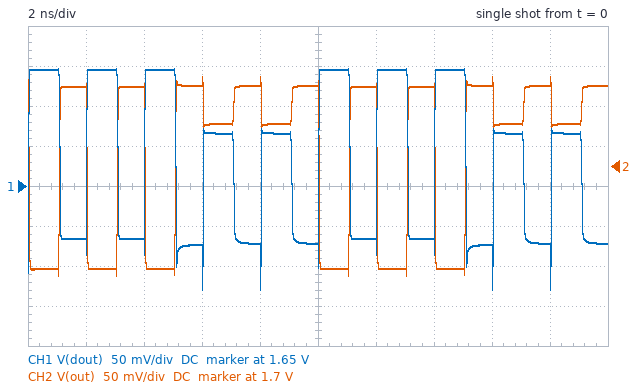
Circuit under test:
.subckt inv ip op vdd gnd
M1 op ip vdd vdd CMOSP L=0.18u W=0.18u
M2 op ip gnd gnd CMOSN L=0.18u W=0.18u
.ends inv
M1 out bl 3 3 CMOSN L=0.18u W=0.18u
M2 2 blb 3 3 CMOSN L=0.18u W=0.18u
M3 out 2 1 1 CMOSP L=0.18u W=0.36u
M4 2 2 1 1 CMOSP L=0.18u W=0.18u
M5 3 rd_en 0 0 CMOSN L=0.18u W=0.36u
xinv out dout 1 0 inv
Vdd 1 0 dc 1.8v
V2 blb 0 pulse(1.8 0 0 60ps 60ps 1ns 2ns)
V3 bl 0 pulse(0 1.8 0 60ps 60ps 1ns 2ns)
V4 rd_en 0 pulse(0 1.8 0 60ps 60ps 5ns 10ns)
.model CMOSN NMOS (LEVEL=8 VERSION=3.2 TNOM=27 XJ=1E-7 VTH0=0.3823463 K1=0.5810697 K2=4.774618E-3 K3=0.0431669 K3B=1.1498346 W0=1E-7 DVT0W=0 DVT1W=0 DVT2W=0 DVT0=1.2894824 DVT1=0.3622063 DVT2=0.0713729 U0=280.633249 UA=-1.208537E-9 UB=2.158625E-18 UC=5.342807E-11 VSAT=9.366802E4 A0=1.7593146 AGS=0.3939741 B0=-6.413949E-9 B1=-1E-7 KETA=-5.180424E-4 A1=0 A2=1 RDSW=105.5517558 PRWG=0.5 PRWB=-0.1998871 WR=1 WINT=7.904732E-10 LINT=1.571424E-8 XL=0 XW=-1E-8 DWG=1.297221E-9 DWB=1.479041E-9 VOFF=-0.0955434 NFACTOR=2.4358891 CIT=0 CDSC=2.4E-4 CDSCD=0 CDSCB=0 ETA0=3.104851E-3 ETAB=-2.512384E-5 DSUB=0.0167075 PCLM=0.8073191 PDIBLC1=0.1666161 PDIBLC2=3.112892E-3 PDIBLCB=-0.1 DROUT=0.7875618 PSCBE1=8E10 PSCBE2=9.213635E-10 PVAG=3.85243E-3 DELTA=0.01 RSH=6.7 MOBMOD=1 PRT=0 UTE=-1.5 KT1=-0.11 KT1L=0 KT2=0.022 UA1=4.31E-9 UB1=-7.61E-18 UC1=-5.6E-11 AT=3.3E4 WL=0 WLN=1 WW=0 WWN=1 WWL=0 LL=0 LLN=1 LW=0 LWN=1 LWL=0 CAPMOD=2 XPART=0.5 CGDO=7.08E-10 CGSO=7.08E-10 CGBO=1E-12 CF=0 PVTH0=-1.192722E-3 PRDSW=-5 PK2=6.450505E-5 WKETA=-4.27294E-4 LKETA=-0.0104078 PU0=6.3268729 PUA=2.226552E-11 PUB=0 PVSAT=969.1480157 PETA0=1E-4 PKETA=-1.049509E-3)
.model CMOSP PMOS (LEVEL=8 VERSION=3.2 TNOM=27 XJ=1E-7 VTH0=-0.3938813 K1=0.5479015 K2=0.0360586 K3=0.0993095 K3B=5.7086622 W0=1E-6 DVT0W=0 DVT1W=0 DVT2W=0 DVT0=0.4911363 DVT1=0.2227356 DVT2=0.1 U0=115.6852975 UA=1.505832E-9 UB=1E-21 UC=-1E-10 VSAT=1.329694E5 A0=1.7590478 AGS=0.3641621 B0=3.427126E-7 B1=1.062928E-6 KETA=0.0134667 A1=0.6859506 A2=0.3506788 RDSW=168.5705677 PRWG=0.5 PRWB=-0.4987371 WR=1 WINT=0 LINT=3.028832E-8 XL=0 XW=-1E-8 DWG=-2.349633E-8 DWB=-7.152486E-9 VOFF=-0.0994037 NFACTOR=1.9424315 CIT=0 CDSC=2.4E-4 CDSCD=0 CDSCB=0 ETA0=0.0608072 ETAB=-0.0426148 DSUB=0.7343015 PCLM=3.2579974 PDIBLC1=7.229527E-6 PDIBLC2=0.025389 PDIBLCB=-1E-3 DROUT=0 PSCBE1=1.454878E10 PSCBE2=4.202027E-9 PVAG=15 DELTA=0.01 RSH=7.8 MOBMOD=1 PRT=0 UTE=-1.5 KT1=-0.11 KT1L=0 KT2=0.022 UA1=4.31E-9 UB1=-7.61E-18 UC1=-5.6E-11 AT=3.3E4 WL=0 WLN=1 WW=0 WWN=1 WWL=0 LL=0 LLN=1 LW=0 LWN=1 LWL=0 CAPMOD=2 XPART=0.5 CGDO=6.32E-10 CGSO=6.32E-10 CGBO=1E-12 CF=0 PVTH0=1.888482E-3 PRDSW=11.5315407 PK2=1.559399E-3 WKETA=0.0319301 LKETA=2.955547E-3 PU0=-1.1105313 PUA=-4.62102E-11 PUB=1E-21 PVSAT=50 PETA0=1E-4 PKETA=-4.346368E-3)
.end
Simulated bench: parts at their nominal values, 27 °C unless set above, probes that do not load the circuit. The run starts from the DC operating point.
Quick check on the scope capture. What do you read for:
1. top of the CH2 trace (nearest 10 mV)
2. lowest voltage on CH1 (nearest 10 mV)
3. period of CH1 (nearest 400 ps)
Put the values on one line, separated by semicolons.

1.81 V; 1.52 V; 2.0 ns
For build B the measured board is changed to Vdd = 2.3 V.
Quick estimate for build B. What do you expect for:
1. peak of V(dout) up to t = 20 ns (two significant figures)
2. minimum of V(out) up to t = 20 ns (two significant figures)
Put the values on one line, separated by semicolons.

2.3 V; 2.1 V
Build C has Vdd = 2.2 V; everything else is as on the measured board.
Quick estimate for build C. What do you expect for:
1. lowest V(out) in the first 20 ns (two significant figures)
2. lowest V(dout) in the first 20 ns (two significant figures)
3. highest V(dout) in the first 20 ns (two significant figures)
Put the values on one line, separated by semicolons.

2.0 V; 1.9 V; 2.2 V
